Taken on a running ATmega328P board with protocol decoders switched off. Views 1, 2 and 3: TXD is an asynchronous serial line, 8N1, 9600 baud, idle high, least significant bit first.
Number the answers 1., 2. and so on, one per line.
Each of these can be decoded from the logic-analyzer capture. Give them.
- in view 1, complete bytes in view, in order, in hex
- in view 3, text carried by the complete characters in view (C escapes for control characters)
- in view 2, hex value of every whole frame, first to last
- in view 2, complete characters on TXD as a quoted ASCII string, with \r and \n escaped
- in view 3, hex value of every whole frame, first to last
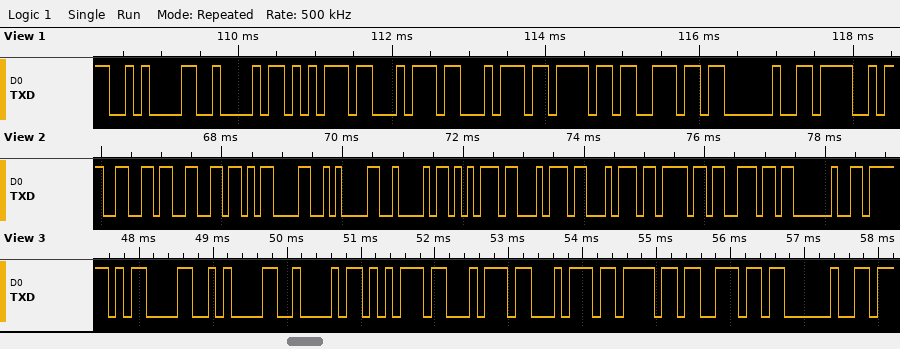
1. 0A 42 75 74 74 6F 6E 20 4F
2. "\r\nButton "
3. 66 66 0D 0A 42 75 74 74 6F 6E 20
4. "ff\r\nButton "
5. 0x0D 0x0A 0x42 0x75 0x74 0x74 0x6F 0x6E 0x20
